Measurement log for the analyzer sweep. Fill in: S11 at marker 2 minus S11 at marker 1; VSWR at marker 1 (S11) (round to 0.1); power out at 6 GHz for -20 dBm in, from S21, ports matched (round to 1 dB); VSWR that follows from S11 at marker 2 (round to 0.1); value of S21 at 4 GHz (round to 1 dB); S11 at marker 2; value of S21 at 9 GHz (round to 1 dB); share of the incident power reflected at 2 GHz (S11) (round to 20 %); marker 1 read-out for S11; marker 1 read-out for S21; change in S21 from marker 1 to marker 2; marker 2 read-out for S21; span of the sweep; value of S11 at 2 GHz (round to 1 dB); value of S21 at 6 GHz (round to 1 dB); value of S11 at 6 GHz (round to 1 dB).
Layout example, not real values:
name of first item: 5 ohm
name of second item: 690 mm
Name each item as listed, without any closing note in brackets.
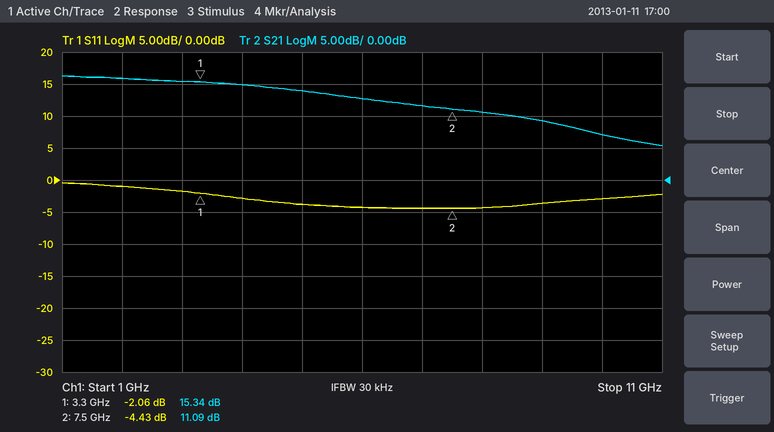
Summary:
S11 at marker 2 minus S11 at marker 1: -2.37 dB
VSWR at marker 1 (S11): 8.5
power out at 6 GHz for -20 dBm in, from S21, ports matched: -7 dBm
VSWR that follows from S11 at marker 2: 4.0
value of S21 at 4 GHz: 15 dB
S11 at marker 2: -4.43 dB
value of S21 at 9 GHz: 9 dB
share of the incident power reflected at 2 GHz (S11): 80 %
marker 1 read-out for S11: -2.06 dB
marker 1 read-out for S21: 15.34 dB
change in S21 from marker 1 to marker 2: -4.25 dB
marker 2 read-out for S21: 11.09 dB
span of the sweep: 10 GHz
value of S11 at 2 GHz: -1 dB
value of S21 at 6 GHz: 13 dB
value of S11 at 6 GHz: -4 dB
